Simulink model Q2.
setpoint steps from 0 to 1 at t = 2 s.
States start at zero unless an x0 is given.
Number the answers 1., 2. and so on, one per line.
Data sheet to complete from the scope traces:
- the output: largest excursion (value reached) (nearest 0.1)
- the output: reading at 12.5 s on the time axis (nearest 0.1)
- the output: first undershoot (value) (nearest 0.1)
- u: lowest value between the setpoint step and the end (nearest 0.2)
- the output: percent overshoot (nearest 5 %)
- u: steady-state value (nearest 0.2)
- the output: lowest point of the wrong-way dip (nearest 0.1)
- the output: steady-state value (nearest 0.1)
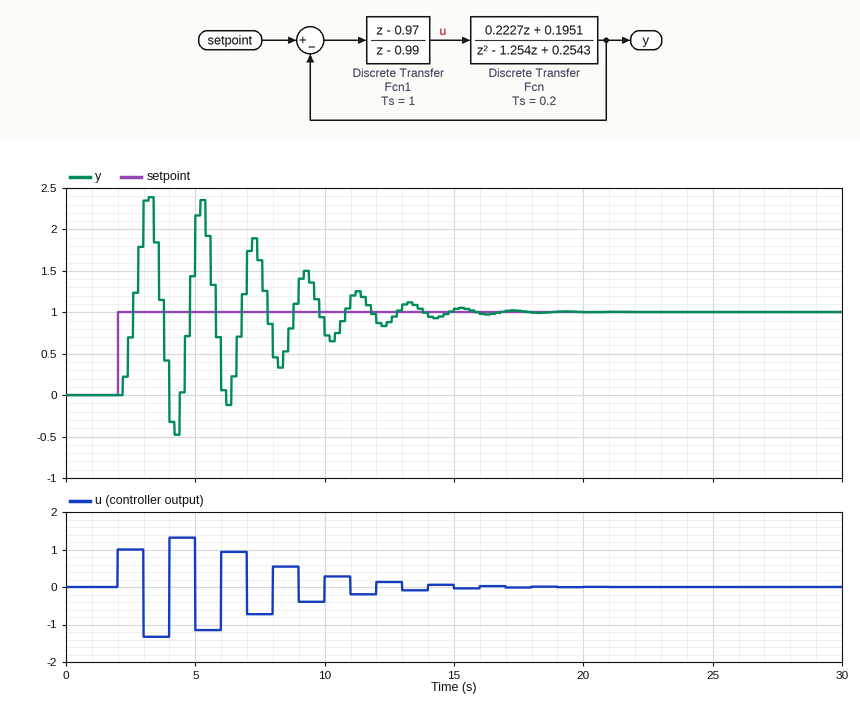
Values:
1. 2.4
2. 0.9
3. -0.5
4. -1.4
5. 140 %
6. 0.0
7. -0.5
8. 1.0
